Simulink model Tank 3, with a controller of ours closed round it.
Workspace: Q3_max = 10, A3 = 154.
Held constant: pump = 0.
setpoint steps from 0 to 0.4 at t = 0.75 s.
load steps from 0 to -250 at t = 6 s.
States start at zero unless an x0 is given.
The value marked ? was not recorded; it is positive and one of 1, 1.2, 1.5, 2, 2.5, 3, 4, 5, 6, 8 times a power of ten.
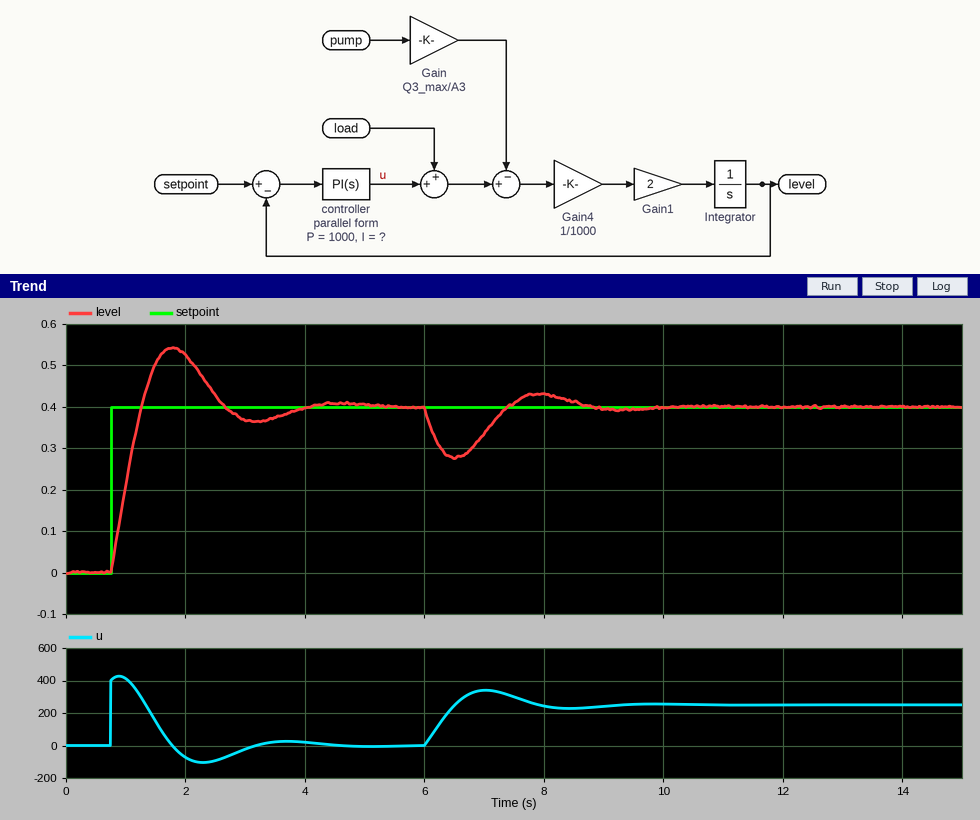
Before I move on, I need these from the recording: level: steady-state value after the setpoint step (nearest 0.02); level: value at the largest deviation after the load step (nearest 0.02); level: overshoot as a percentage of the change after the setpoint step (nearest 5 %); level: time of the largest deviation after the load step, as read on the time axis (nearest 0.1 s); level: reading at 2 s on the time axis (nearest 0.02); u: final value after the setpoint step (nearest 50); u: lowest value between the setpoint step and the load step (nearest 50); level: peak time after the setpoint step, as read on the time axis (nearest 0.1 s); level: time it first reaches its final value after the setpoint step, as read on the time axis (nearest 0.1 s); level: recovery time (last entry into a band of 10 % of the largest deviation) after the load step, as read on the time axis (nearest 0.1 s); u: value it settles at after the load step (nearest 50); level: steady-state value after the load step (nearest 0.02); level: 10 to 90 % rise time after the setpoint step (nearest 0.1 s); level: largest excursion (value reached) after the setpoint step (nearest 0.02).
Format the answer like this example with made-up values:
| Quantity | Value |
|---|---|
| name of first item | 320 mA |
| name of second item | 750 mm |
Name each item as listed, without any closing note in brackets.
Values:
| Quantity | Value |
|---|---|
| level: steady-state value after the setpoint step | 0.40 |
| level: value at the largest deviation after the load step | 0.28 |
| level: overshoot as a percentage of the change after the setpoint step | 35 % |
| level: time of the largest deviation after the load step, as read on the time axis | 6.5 s |
| level: reading at 2 s on the time axis | 0.52 |
| u: final value after the setpoint step | 0 |
| u: lowest value between the setpoint step and the load step | -100 |
| level: peak time after the setpoint step, as read on the time axis | 1.8 s |
| level: time it first reaches its final value after the setpoint step, as read on the time axis | 1.3 s |
| level: recovery time (last entry into a band of 10 % of the largest deviation) after the load step, as read on the time axis | 8.5 s |
| u: value it settles at after the load step | 250 |
| level: steady-state value after the load step | 0.40 |
| level: 10 to 90 % rise time after the setpoint step | 0.4 s |
| level: largest excursion (value reached) after the setpoint step | 0.54 |
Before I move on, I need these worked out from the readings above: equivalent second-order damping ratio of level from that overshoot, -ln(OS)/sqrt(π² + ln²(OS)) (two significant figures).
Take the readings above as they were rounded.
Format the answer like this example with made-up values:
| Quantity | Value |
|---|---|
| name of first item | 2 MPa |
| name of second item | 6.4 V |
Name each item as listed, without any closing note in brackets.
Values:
| Quantity | Value |
|---|---|
| equivalent second-order damping ratio of level from that overshoot, -ln(OS)/sqrt(π² + ln²(OS)) | 0.32 |
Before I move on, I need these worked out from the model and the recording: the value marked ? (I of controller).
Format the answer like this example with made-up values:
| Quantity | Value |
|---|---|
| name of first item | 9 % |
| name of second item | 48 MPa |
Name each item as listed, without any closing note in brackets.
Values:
| Quantity | Value |
|---|---|
| the value marked ? | 3000 |
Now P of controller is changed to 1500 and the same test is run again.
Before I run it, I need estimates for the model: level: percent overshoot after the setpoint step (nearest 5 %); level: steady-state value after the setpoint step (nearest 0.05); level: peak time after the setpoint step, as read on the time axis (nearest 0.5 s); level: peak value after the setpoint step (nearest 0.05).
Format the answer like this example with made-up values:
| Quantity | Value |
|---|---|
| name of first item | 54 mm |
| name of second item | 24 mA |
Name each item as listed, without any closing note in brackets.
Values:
| Quantity | Value |
|---|---|
| level: percent overshoot after the setpoint step | 25 % |
| level: steady-state value after the setpoint step | 0.40 |
| level: peak time after the setpoint step, as read on the time axis | 1.5 s |
| level: peak value after the setpoint step | 0.50 |
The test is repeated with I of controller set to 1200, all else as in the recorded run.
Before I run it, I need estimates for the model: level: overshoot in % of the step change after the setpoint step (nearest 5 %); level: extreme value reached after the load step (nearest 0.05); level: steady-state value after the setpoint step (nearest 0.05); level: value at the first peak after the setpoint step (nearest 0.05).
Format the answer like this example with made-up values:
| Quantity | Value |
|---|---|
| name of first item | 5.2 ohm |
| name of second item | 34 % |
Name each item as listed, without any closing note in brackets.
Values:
| Quantity | Value |
|---|---|
| level: overshoot in % of the step change after the setpoint step | 25 % |
| level: extreme value reached after the load step | 0.25 |
| level: steady-state value after the setpoint step | 0.40 |
| level: value at the first peak after the setpoint step | 0.50 |
